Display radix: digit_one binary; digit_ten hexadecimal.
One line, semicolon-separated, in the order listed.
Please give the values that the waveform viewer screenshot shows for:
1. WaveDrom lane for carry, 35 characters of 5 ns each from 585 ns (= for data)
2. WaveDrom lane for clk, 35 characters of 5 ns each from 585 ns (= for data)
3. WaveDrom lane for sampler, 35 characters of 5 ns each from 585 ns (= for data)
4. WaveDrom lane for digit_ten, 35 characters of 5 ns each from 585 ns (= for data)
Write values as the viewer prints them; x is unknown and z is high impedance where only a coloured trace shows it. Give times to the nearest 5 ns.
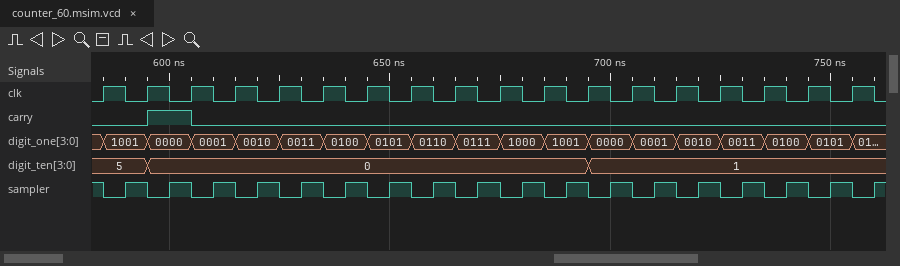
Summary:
{name: 'carry', wave: '0.1.0..............................'}; {name: 'clk', wave: '10101010101010101010101010101010101'}; {name: 'sampler', wave: '01010101010101010101010101010101010'}; {name: 'digit_ten', wave: '=.=...................=............', data: '5 0 1'}
